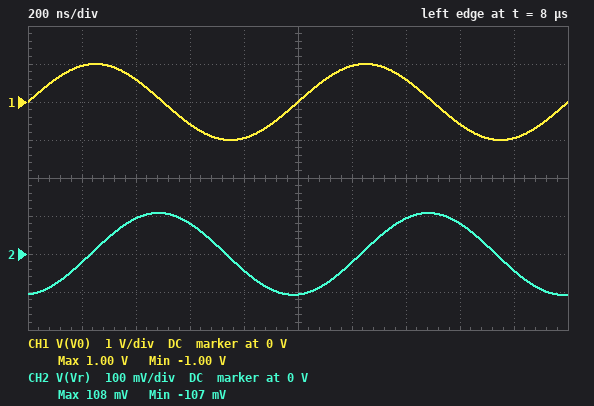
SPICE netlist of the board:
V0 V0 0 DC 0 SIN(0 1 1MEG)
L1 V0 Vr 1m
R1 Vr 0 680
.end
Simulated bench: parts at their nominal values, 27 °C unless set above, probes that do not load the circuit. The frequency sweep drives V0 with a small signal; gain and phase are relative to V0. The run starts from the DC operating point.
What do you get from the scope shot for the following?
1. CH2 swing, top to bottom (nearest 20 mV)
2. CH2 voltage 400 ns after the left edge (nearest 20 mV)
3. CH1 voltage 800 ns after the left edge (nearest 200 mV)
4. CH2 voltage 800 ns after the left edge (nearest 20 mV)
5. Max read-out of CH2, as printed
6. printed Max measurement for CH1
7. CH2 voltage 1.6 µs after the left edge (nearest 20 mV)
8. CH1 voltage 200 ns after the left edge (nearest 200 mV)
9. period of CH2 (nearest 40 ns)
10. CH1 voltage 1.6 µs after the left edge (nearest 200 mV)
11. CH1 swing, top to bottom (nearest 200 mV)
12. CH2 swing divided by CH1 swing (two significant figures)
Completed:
220 mV
100 mV
-1.0 V
-40 mV
108 mV
1.00 V
80 mV
1.0 V
1.00 µs
-600 mV
2.0 V
0.11
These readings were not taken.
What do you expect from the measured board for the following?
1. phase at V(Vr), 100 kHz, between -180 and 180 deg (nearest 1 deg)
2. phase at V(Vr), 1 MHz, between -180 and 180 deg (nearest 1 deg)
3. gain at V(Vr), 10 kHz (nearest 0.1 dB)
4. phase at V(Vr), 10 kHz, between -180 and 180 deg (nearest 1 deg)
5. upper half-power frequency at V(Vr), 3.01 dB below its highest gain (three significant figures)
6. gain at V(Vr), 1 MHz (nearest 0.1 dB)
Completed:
-43 deg
-84 deg
0 dB
-5 deg
108 kHz
-19.4 dB
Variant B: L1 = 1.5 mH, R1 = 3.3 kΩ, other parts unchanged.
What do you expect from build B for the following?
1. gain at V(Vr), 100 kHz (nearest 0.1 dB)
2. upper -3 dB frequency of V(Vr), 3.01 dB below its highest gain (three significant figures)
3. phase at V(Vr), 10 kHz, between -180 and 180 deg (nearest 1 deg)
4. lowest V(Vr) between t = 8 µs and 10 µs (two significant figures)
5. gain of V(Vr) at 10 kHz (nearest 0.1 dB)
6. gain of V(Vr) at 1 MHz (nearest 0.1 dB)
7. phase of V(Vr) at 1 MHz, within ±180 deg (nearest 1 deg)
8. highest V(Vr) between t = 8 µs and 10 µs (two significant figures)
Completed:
-0.3 dB
350 kHz
-2 deg
-330 mV
0 dB
-9.6 dB
-71 deg
330 mV
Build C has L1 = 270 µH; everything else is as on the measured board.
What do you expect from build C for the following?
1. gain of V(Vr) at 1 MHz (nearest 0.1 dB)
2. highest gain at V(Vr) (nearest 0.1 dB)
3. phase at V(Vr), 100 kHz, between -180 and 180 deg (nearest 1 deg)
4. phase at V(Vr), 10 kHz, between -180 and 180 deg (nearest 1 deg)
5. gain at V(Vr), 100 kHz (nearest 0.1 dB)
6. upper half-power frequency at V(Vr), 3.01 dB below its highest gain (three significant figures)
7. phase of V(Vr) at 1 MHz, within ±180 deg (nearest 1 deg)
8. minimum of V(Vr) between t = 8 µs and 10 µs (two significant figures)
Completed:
-8.6 dB
0 dB
-14 deg
-1 deg
-0.3 dB
401 kHz
-68 deg
-370 mV
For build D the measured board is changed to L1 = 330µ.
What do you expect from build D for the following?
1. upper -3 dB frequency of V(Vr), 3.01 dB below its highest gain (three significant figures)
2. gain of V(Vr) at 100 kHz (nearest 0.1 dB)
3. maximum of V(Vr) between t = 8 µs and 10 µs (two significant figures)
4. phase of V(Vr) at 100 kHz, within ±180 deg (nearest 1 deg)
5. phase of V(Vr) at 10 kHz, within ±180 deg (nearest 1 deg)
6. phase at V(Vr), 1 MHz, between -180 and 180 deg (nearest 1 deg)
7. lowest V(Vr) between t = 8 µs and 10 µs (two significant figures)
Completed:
328 kHz
-0.4 dB
310 mV
-17 deg
-2 deg
-72 deg
-310 mV
